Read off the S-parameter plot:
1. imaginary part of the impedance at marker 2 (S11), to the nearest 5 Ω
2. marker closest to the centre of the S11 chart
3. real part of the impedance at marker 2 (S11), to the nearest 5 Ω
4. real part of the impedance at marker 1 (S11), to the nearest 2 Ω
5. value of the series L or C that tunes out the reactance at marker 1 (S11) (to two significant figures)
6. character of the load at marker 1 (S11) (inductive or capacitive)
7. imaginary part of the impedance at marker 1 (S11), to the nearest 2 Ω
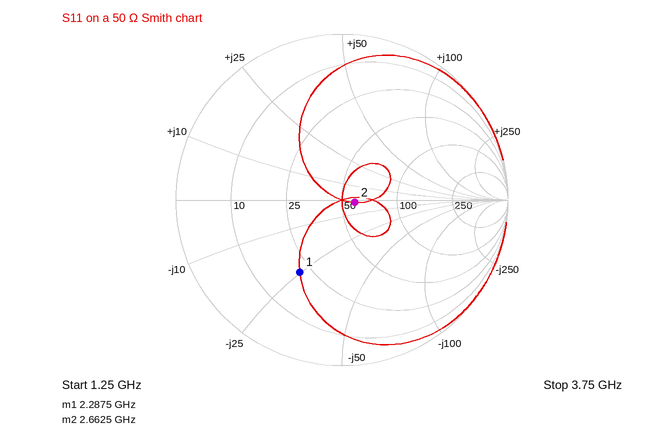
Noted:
0 Ω
marker 2
60 Ω
22 Ω
1.7 nH
capacitive
-24 Ω
